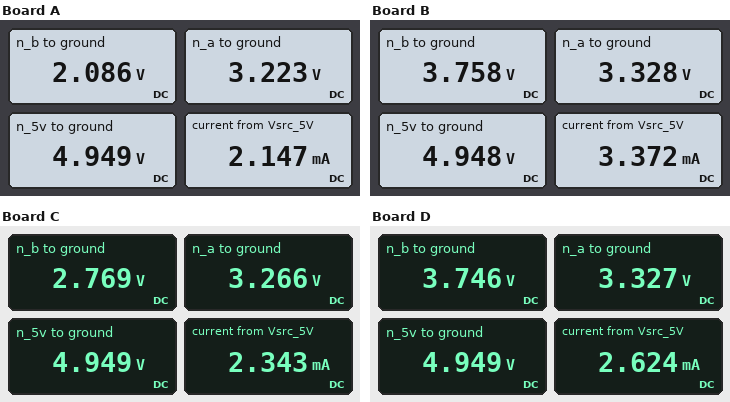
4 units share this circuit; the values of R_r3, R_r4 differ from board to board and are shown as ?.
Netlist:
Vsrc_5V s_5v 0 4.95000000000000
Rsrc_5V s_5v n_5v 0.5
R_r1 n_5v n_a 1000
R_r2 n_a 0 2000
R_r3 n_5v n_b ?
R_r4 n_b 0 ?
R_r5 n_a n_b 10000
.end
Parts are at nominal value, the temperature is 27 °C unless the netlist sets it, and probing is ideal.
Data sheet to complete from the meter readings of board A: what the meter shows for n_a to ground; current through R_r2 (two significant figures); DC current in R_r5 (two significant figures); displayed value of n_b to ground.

3.223 V
1.6 mA
110 µA
2.086 V
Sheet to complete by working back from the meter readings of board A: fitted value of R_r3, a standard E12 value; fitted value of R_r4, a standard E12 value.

6.8 kΩ
3.9 kΩ
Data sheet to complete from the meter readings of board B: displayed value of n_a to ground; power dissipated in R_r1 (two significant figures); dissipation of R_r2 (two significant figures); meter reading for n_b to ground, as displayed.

3.328 V
2.6 mW
5.5 mW
3.758 V
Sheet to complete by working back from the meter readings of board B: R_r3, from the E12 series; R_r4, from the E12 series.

680 Ω
2.2 kΩ
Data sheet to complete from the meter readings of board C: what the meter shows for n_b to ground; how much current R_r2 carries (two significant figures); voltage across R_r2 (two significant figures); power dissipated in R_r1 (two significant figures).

2.769 V
1.6 mA
3.3 V
2.8 mW
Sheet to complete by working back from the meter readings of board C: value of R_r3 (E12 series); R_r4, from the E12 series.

3.3 kΩ
3.9 kΩ
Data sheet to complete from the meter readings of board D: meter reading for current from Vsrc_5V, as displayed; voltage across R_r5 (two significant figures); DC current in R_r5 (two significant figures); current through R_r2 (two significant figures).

2.624 mA
420 mV
42 µA
1.7 mA
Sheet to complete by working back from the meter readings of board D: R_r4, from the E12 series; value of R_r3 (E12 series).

3.9 kΩ
1.2 kΩ
